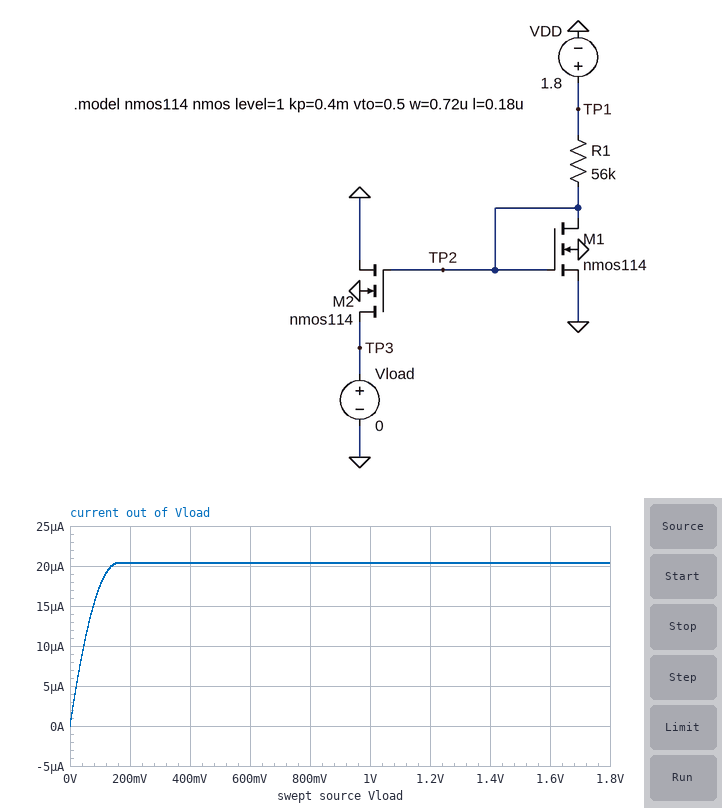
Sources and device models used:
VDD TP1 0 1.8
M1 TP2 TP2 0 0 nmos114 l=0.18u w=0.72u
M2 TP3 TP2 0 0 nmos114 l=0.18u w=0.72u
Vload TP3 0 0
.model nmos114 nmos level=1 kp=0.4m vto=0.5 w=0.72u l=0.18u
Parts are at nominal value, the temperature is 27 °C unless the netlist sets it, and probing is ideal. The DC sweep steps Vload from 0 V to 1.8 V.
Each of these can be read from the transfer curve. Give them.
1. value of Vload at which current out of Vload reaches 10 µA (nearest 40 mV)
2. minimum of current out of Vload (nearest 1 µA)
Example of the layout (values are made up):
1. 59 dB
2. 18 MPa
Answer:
1. 40 mV
2. 0 A
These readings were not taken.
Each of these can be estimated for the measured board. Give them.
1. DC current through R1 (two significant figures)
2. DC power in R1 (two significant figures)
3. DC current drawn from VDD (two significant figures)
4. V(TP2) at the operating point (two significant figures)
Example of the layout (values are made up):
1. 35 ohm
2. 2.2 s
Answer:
1. 20 µA
2. 23 µW
3. 20 µA
4. 660 mV
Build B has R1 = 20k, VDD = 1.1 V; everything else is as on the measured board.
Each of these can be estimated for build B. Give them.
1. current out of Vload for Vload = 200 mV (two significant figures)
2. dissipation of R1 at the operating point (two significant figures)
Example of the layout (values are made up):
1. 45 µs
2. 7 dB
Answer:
1. 22 µA
2. 9.5 µW
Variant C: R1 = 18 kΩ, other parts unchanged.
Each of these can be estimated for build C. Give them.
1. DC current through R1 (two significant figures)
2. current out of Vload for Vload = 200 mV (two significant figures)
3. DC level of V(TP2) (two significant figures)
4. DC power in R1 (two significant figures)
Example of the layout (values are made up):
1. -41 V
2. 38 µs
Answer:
1. 57 µA
2. 54 µA
3. 770 mV
4. 59 µW
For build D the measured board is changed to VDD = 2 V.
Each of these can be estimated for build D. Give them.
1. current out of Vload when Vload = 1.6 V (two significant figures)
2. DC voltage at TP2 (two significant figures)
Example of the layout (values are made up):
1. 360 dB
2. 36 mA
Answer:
1. 24 µA
2. 670 mV
